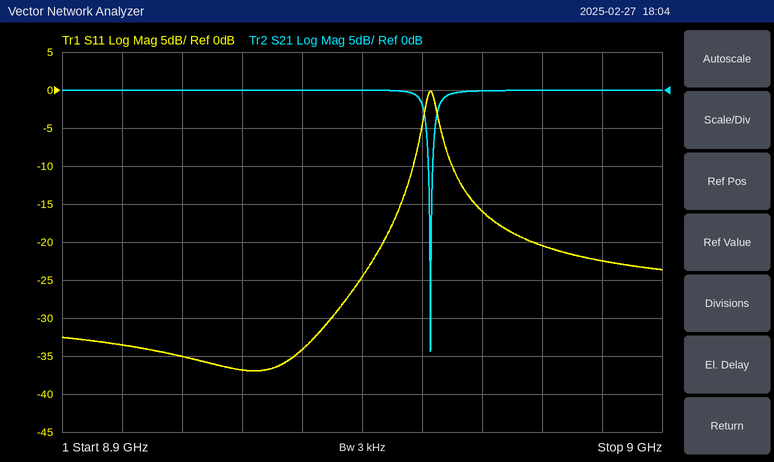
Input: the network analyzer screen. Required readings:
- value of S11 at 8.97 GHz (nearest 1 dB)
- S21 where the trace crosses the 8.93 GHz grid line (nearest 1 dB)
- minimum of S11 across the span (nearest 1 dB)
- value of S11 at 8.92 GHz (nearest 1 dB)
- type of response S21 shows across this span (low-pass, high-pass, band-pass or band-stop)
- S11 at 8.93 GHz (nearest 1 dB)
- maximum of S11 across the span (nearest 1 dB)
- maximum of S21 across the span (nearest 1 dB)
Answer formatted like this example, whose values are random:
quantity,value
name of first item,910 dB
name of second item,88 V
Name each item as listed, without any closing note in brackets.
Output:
quantity,value
value of S11 at 8.97 GHz,-16 dB
S21 where the trace crosses the 8.93 GHz grid line,0 dB
minimum of S11 across the span,-37 dB
value of S11 at 8.92 GHz,-35 dB
type of response S21 shows across this span,band-stop
S11 at 8.93 GHz,-37 dB
maximum of S11 across the span,0 dB
maximum of S21 across the span,0 dB
